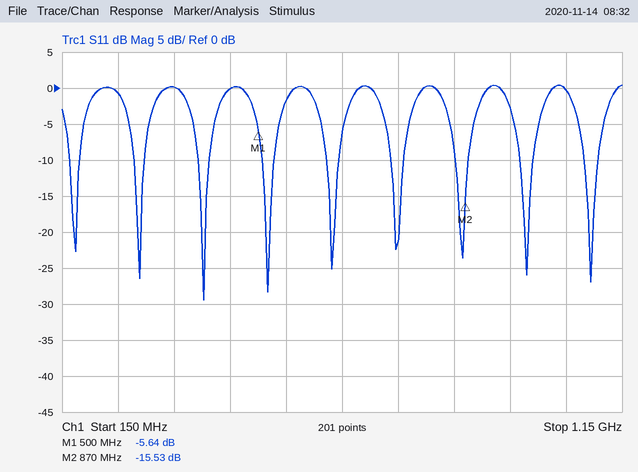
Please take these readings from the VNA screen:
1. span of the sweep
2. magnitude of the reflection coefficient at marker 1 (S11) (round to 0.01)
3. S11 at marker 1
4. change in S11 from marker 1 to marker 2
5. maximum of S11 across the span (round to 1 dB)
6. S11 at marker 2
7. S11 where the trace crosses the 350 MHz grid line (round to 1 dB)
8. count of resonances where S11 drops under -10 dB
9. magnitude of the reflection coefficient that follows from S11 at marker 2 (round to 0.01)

1 GHz
0.52
-5.64 dB
-9.89 dB
0 dB
-15.53 dB
0 dB
9
0.17
